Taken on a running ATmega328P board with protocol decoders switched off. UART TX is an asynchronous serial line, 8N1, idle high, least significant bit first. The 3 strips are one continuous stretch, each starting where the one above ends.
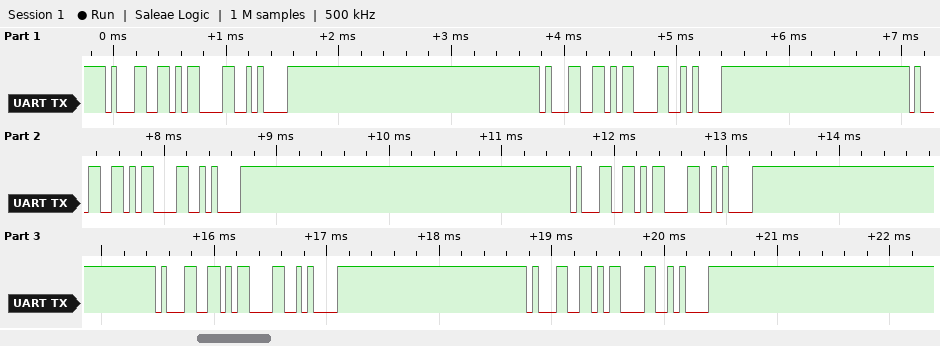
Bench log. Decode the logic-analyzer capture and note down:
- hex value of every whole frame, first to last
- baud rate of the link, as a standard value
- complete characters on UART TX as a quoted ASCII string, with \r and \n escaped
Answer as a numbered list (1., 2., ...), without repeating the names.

1. 0x31 0x0D 0x0A 0x31 0x0D 0x0A 0x31 0x0D 0x0A 0x31 0x0D 0x0A 0x31 0x0D 0x0A 0x31 0x0D 0x0A
2. 19200 baud
3. "1\r\n1\r\n1\r\n1\r\n1\r\n1\r\n"
